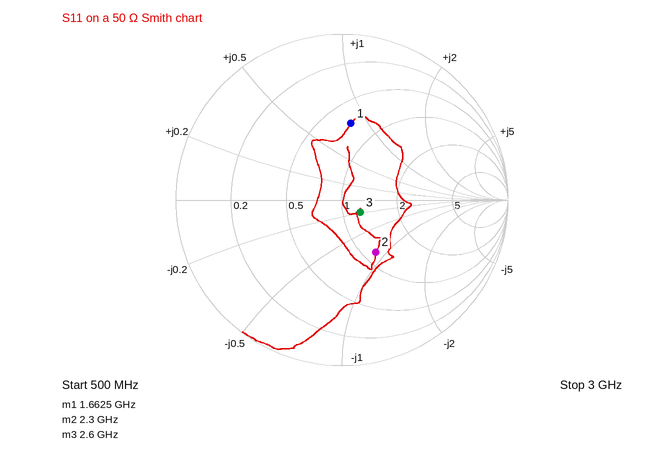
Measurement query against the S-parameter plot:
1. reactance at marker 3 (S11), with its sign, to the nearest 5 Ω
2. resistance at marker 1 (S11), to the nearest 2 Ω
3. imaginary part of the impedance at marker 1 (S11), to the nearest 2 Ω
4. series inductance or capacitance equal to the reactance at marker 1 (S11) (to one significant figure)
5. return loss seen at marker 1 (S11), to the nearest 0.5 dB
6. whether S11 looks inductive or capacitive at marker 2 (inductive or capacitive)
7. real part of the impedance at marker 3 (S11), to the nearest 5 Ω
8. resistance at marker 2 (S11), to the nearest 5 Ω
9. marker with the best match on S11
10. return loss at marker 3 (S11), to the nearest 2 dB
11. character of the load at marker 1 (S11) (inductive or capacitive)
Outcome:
-10 Ω
36 Ω
+42 Ω
4 nH
6.5 dB
capacitive
60 Ω
60 Ω
marker 3
18 dB
inductive
